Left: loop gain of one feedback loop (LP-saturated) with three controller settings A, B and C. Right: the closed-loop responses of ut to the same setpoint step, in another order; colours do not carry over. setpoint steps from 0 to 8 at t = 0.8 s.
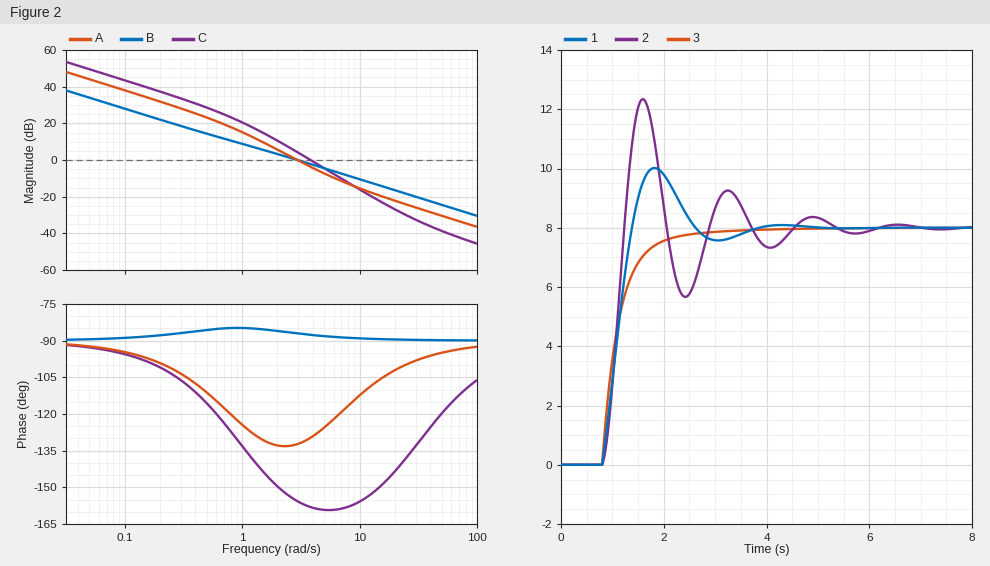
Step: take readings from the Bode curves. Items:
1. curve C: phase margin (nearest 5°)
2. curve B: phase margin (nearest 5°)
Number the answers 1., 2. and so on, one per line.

1. 20°
2. 95°
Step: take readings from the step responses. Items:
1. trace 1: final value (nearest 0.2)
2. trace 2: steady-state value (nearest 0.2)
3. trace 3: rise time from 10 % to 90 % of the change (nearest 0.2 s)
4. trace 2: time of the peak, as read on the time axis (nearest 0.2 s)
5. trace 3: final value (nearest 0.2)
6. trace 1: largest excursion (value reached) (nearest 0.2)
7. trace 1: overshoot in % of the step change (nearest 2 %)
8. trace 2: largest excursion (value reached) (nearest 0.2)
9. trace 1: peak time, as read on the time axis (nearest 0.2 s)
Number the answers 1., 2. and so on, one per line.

1. 8.0
2. 8.0
3. 0.8 s
4. 1.6 s
5. 8.0
6. 10.0
7. 26 %
8. 12.4
9. 1.8 s
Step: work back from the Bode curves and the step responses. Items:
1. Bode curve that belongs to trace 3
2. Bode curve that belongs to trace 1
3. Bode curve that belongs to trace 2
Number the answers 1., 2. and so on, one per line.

1. B
2. A
3. C
